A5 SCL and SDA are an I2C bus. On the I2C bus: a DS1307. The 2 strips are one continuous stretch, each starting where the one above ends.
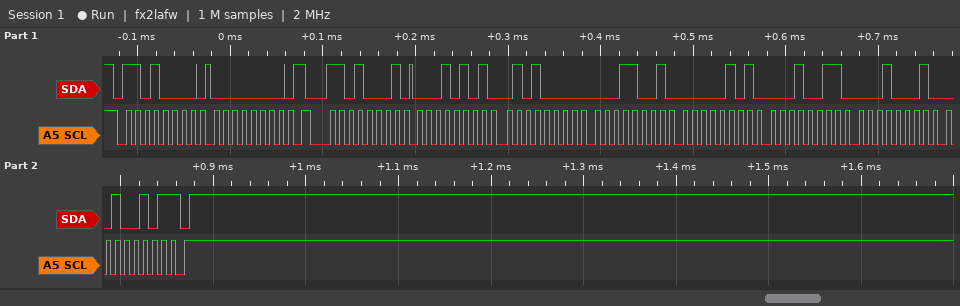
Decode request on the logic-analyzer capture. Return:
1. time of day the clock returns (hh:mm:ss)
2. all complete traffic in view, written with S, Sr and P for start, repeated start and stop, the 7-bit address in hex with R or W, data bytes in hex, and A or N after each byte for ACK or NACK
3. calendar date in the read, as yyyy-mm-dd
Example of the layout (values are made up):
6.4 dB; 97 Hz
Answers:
19:50:15; S 68W A 00 A Sr 68R A 15 A 50 A 19 A 05 A 13 A 11 A 25 N P; 2025-11-13
